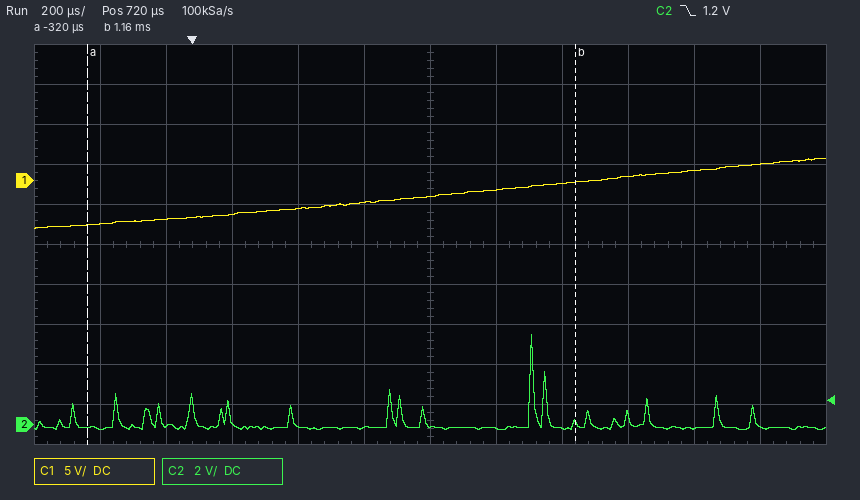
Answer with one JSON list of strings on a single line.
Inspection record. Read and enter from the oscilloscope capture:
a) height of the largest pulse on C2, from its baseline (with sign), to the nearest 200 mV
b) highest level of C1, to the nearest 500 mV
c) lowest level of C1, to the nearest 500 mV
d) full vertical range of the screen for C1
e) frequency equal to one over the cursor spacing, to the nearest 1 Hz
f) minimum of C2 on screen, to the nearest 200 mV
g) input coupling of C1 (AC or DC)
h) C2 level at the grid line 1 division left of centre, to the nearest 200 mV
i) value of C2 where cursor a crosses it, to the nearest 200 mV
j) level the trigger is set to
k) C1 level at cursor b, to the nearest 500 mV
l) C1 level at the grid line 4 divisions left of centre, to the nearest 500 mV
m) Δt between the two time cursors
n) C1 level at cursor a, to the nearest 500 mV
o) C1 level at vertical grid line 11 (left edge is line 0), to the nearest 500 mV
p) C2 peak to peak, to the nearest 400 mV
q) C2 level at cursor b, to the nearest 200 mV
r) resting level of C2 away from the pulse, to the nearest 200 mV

["+4.6 V", "2.5 V", "-6.0 V", "50 V", "676 Hz", "-200 mV", "DC", "-200 mV", "-200 mV", "1.2 V", "0.0 V", "-5.0 V", "1.48 ms", "-5.5 V", "2.0 V", "4.8 V", "0.0 V", "-200 mV"]
